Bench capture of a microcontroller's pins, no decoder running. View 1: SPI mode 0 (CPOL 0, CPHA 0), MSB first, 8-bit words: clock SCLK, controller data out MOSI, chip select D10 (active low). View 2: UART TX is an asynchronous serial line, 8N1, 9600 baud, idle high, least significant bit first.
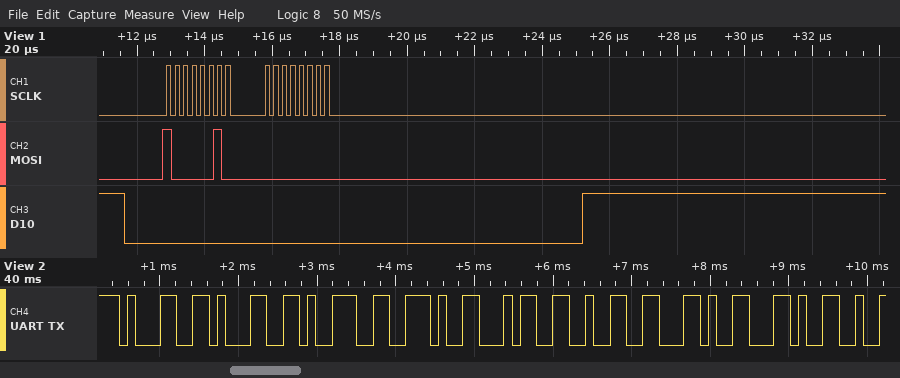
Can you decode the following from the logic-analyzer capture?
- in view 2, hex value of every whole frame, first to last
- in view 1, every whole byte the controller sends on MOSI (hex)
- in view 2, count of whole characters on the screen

31 31 39 2E 34 32 2C 2C
82 00
8
